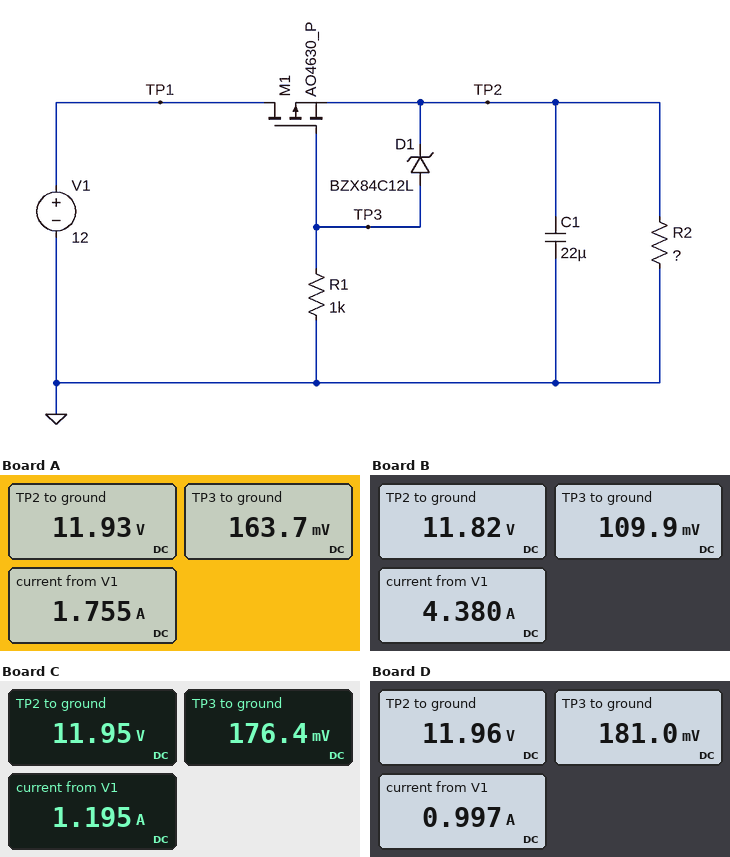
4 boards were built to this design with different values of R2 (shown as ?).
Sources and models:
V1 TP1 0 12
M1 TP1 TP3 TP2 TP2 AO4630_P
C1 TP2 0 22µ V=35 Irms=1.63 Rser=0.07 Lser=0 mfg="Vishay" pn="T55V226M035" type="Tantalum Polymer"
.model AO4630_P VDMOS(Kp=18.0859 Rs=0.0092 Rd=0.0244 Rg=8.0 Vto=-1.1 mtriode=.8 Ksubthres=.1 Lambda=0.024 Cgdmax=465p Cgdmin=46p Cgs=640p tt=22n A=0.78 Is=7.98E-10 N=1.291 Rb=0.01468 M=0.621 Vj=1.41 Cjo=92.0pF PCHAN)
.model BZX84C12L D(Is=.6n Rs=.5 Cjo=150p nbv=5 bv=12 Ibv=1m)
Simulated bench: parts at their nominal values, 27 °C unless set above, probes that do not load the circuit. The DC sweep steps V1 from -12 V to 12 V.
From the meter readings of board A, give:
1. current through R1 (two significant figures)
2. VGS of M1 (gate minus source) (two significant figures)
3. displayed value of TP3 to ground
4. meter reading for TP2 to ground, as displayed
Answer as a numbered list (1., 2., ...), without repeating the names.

1. 160 µA
2. -12 V
3. 163.7 mV
4. 11.93 V
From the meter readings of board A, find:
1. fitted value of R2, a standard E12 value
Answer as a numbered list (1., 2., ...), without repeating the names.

1. 6.8 Ω
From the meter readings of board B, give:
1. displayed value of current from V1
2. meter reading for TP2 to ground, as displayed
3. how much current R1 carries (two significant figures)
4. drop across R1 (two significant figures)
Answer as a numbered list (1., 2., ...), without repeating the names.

1. 4.380 A
2. 11.82 V
3. 110 µA
4. 110 mV
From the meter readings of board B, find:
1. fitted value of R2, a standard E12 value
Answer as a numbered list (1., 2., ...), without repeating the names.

1. 2.7 Ω
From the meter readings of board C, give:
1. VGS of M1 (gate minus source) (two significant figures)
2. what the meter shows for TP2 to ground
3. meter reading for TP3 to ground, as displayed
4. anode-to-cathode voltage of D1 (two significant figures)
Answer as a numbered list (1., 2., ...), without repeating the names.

1. -12 V
2. 11.95 V
3. 176.4 mV
4. -12 V
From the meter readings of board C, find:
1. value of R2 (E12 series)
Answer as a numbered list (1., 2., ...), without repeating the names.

1. 10 Ω
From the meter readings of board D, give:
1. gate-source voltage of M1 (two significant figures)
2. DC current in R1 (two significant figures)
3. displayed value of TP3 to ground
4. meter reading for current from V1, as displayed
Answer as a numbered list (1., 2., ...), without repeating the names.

1. -12 V
2. 180 µA
3. 181.0 mV
4. 0.997 A
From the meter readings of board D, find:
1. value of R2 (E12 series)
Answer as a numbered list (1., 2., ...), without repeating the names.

1. 12 Ω
